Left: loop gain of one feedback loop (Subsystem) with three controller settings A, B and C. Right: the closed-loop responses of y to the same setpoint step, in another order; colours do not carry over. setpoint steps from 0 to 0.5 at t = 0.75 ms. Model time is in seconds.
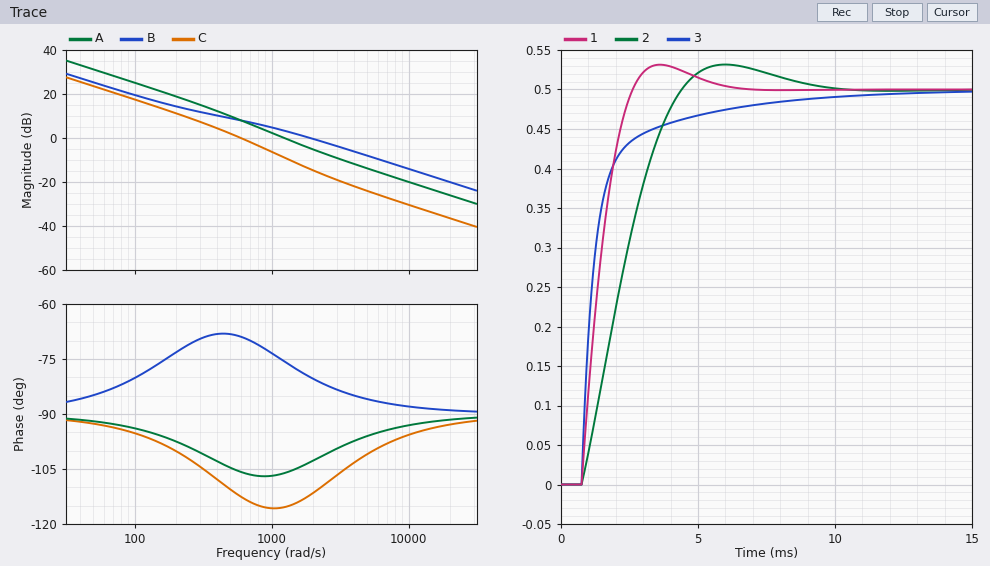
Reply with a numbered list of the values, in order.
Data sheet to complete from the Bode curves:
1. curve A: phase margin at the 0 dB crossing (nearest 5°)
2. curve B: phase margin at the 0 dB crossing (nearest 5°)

1. 75°
2. 100°
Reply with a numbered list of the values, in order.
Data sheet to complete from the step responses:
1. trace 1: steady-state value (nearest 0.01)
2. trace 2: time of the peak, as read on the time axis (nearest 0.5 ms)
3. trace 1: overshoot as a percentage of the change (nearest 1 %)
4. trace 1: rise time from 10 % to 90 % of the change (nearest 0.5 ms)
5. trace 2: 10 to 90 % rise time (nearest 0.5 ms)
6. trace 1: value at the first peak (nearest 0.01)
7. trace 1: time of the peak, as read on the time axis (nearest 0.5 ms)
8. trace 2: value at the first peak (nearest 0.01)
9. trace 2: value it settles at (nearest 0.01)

1. 0.50
2. 6.0 ms
3. 6 %
4. 1.5 ms
5. 2.5 ms
6. 0.53
7. 3.5 ms
8. 0.53
9. 0.50
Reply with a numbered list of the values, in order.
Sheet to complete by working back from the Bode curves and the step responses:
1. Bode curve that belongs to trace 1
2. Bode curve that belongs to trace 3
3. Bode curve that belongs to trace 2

1. A
2. B
3. C
